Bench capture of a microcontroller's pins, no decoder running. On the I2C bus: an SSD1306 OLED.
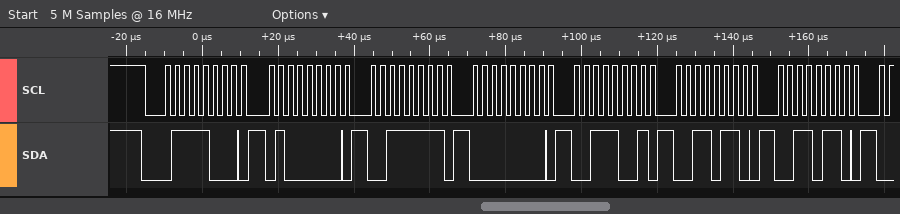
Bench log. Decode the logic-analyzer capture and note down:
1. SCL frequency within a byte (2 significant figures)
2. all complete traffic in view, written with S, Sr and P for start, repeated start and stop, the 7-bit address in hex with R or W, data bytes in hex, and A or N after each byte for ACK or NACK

400 kHz
S 3CW A 40 A 3F A 00 A 39 A 36 A 36 A
